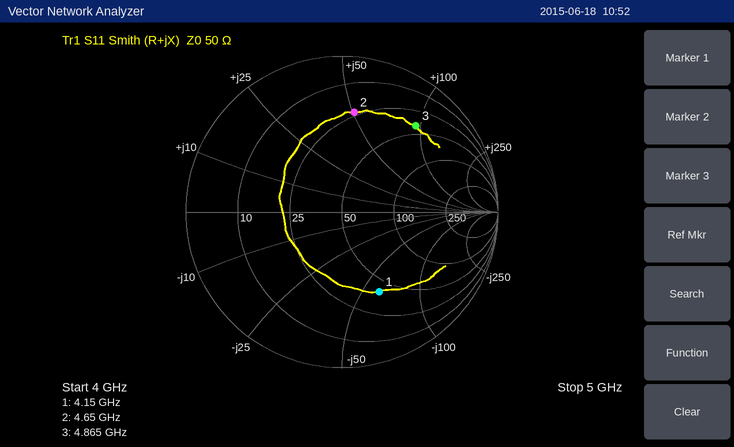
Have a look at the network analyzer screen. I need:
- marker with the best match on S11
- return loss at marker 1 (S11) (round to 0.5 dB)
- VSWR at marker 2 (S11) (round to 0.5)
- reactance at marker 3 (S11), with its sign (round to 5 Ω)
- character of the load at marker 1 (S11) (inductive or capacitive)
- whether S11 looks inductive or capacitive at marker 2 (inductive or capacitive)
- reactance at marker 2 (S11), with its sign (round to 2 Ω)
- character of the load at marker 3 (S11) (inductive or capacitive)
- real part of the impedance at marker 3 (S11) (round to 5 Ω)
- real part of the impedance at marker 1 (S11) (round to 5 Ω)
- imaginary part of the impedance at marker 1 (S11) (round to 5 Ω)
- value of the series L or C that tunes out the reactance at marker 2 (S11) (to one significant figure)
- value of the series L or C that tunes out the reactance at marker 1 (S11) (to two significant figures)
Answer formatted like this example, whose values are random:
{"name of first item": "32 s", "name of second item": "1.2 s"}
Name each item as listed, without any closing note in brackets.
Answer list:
{"marker with the best match on S11": "marker 1", "return loss at marker 1 (S11)": "5.0 dB", "VSWR at marker 2 (S11)": "4.5", "reactance at marker 3 (S11), with its sign": "+95 Ω", "character of the load at marker 1 (S11)": "capacitive", "whether S11 looks inductive or capacitive at marker 2": "inductive", "reactance at marker 2 (S11), with its sign": "+50 Ω", "character of the load at marker 3 (S11)": "inductive", "real part of the impedance at marker 3 (S11)": "40 Ω", "real part of the impedance at marker 1 (S11)": "40 Ω", "imaginary part of the impedance at marker 1 (S11)": "-60 Ω", "value of the series L or C that tunes out the reactance at marker 2 (S11)": "700 fF", "value of the series L or C that tunes out the reactance at marker 1 (S11)": "2.3 nH"}
